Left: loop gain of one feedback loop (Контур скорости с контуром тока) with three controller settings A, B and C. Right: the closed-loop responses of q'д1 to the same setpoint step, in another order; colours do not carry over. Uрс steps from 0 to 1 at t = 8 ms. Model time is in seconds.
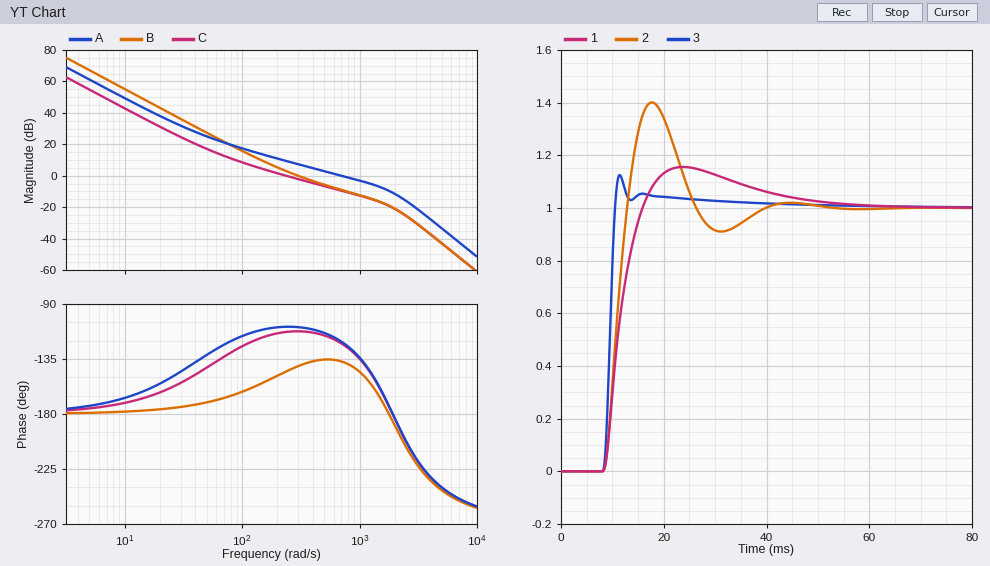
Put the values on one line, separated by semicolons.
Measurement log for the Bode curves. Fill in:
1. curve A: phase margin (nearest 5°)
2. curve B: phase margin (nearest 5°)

60°; 40°
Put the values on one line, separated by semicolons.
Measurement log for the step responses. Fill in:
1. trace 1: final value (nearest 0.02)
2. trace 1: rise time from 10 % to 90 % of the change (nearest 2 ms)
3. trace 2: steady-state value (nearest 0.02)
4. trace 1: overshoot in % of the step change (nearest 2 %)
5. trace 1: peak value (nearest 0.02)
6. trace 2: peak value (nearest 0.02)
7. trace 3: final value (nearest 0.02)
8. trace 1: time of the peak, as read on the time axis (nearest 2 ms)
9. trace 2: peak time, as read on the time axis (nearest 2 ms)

1.00; 6 ms; 1.00; 16 %; 1.16; 1.40; 1.00; 24 ms; 18 ms
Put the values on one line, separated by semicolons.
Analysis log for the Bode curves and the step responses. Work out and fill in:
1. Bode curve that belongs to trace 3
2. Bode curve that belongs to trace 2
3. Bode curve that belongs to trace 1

A; B; C
